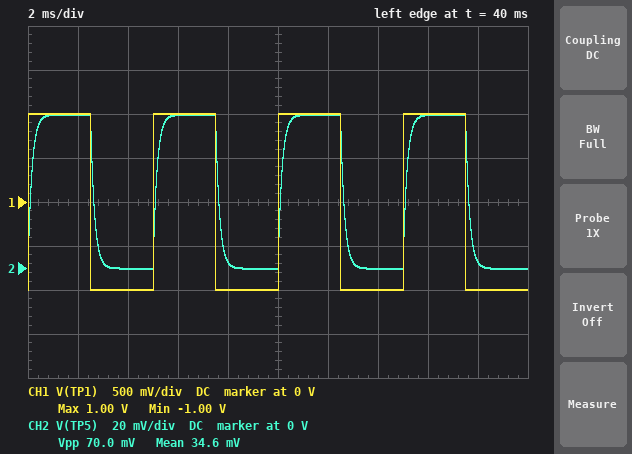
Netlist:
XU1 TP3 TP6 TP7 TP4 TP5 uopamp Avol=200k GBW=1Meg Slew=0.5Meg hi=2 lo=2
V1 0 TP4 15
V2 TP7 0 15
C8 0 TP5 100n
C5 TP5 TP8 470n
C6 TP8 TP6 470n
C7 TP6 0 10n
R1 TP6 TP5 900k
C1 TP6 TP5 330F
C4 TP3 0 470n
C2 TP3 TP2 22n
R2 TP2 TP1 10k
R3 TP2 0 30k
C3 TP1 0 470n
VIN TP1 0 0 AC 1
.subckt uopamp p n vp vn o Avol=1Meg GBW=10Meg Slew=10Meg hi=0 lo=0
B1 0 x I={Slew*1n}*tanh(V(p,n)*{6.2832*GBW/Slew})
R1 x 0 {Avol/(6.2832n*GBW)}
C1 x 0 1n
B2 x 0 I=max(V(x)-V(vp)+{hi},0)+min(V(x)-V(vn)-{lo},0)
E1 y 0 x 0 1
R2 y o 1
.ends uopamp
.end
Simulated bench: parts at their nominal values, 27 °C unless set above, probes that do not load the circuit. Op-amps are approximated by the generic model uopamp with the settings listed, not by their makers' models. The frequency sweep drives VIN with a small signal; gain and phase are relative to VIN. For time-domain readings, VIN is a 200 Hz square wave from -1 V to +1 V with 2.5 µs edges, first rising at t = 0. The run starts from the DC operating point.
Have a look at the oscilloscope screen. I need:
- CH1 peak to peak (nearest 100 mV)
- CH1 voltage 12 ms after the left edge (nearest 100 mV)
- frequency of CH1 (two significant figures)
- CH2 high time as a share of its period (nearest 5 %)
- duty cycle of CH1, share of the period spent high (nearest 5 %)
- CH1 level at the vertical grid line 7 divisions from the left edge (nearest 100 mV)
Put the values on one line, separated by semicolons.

2.0 V; 1.0 V; 200 Hz; 50 %; 50 %; -1.0 V
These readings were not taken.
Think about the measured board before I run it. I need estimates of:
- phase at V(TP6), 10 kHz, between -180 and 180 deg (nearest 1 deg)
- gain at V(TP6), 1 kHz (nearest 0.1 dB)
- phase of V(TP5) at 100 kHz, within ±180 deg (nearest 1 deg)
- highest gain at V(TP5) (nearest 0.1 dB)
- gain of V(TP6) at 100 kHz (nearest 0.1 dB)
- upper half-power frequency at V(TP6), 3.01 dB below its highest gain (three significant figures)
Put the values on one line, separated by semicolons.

-85 deg; -32.5 dB; -95 deg; -29.1 dB; -69.4 dB; 1.01 kHz
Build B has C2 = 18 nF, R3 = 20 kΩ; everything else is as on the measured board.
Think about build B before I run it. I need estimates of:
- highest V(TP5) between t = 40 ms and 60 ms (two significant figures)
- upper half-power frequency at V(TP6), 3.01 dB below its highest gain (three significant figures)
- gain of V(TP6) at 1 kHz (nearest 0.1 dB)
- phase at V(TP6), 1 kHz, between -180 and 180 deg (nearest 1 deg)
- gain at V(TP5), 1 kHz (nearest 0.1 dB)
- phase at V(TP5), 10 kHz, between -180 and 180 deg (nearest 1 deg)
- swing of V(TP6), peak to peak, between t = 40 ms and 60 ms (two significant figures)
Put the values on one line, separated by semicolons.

51 mV; 1.38 kHz; -34.0 dB; -36 deg; -33.7 dB; -83 deg; 49 mV
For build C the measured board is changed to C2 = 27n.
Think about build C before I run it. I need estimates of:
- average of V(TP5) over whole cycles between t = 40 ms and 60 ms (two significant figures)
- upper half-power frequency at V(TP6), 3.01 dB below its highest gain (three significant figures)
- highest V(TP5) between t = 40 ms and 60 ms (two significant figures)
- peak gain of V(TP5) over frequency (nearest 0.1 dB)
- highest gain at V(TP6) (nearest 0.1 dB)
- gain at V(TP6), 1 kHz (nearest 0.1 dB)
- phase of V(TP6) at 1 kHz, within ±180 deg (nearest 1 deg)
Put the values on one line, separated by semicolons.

42 mV; 831 Hz; 85 mV; -27.4 dB; -27.8 dB; -31.7 dB; -50 deg
